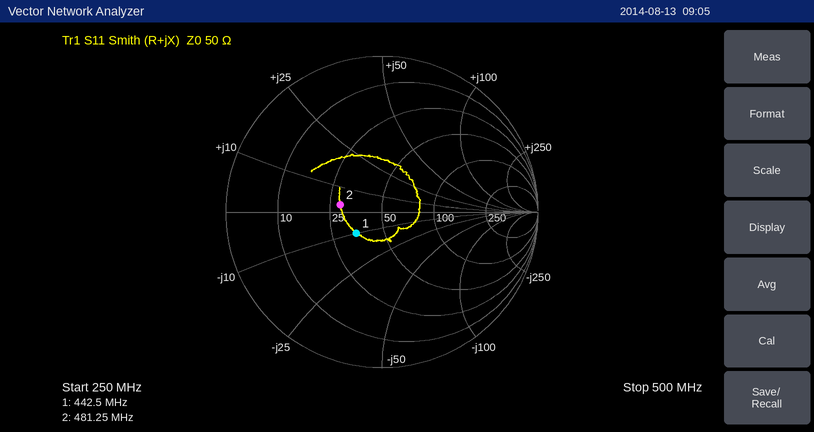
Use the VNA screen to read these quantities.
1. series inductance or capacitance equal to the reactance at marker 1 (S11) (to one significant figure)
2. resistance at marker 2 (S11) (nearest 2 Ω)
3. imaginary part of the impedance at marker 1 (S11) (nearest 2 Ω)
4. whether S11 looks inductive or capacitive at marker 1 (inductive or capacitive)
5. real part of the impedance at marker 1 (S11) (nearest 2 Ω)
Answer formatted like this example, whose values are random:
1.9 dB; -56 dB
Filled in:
40 pF; 28 Ω; -10 Ω; capacitive; 34 Ω
